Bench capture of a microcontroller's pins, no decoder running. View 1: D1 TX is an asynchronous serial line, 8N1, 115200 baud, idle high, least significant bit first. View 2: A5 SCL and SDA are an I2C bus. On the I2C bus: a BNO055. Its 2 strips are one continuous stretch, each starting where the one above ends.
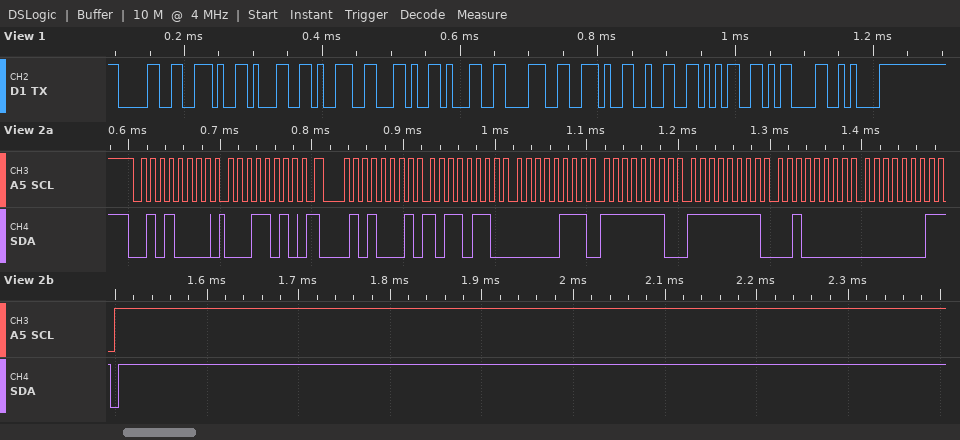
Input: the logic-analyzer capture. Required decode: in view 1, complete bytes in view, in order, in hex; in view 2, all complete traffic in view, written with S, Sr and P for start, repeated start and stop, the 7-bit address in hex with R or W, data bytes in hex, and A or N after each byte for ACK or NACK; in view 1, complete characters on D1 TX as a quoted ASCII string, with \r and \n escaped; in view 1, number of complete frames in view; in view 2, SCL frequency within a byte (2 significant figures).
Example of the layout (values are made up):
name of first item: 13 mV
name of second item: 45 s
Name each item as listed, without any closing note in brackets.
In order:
in view 1, complete bytes in view, in order, in hex: 30 2E 31 39 2C 31 38 2E 32 35 0D 0A
in view 2, all complete traffic in view, written with S, Sr and P for start, repeated start and stop, the 7-bit address in hex with R or W, data bytes in hex, and A or N after each byte for ACK or NACK: S 28W A 1A A Sr 28R A B6 A 07 A FE A FF A 20 A 01 N P
in view 1, complete characters on D1 TX as a quoted ASCII string, with \r and \n escaped: "0.19,18.25\r\n"
in view 1, number of complete frames in view: 12
in view 2, SCL frequency within a byte: 100 kHz
